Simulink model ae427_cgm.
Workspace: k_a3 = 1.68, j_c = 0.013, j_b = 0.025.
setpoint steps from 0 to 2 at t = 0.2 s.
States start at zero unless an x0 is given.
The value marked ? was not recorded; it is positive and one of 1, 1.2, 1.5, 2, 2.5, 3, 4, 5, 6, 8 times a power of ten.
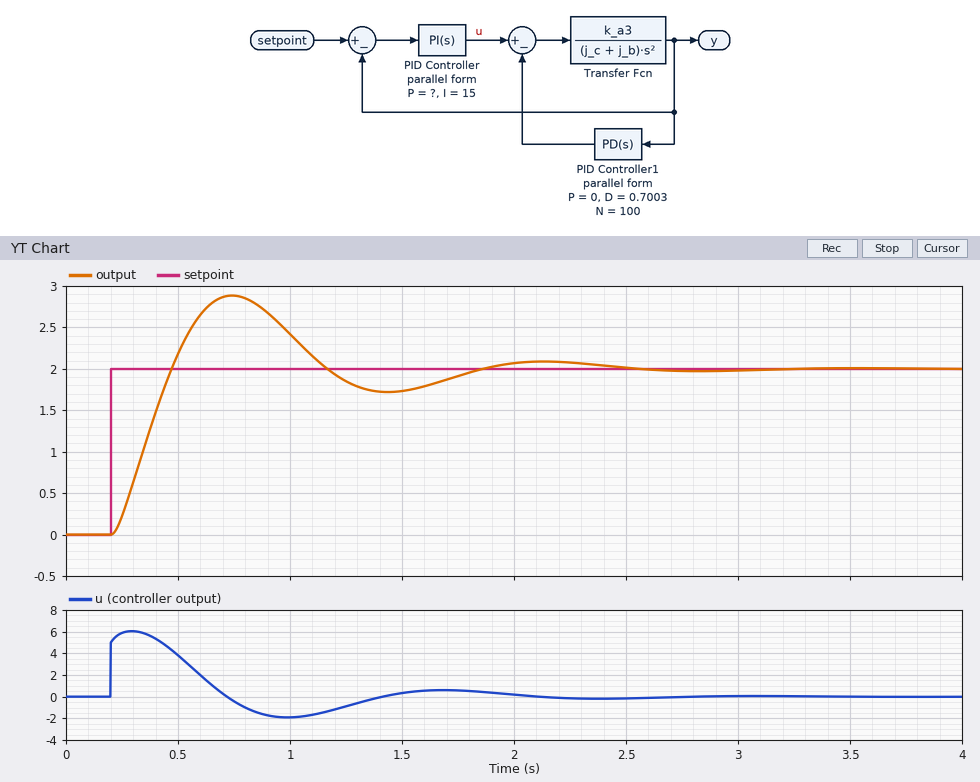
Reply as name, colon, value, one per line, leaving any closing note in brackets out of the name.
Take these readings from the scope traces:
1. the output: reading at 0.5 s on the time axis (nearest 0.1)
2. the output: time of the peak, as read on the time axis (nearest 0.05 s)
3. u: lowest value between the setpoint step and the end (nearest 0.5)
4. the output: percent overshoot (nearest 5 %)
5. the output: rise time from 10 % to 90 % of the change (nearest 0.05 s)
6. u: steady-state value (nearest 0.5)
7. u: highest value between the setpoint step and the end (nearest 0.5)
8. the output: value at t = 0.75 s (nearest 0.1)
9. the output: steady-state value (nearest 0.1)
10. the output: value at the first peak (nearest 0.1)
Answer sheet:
the output: reading at 0.5 s on the time axis: 2.2
the output: time of the peak, as read on the time axis: 0.75 s
u: lowest value between the setpoint step and the end: -2.0
the output: percent overshoot: 45 %
the output: rise time from 10 % to 90 % of the change: 0.20 s
u: steady-state value: 0.0
u: highest value between the setpoint step and the end: 6.0
the output: value at t = 0.75 s: 2.9
the output: steady-state value: 2.0
the output: value at the first peak: 2.9
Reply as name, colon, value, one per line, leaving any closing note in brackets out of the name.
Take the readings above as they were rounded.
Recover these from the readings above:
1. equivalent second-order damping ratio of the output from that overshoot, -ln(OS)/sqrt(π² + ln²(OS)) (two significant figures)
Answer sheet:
equivalent second-order damping ratio of the output from that overshoot, -ln(OS)/sqrt(π² + ln²(OS)): 0.25
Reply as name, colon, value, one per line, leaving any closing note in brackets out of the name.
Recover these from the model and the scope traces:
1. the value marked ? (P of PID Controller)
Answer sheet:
the value marked ?: 2.5
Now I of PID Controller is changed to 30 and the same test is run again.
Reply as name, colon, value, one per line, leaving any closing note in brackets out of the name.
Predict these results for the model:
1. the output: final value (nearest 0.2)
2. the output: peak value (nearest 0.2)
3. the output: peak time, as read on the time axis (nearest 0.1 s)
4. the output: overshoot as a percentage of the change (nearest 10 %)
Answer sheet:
the output: final value: 2.0
the output: peak value: 3.2
the output: peak time, as read on the time axis: 0.6 s
the output: overshoot as a percentage of the change: 60 %
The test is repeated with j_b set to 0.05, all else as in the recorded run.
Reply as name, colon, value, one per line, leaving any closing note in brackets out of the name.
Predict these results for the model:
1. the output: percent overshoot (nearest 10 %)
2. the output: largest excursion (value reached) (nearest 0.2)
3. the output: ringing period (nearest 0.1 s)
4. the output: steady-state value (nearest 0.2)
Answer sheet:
the output: percent overshoot: 50 %
the output: largest excursion (value reached): 3.0
the output: ringing period: 1.3 s
the output: steady-state value: 2.0
